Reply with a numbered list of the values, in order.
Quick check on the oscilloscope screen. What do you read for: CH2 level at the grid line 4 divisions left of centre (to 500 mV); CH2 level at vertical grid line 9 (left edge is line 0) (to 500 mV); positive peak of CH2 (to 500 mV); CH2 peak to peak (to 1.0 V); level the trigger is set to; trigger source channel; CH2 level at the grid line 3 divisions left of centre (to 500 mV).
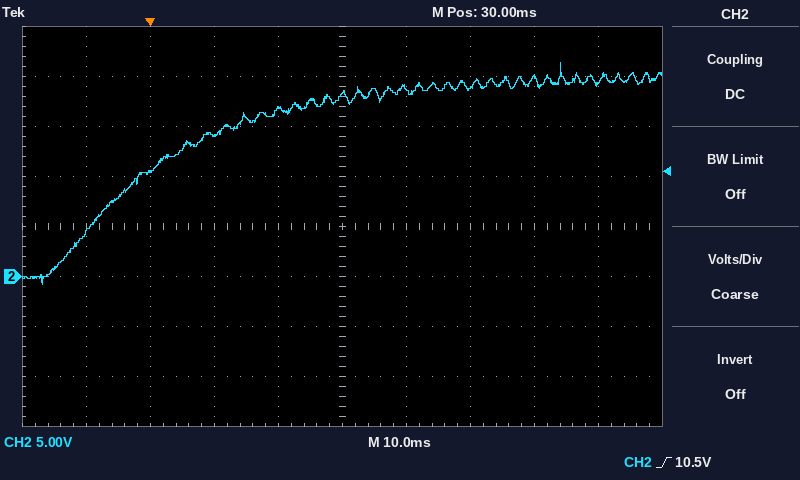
1. 4.5 V
2. 19.5 V
3. 21.5 V
4. 22.0 V
5. 10.5 V
6. CH2
7. 10.5 V
